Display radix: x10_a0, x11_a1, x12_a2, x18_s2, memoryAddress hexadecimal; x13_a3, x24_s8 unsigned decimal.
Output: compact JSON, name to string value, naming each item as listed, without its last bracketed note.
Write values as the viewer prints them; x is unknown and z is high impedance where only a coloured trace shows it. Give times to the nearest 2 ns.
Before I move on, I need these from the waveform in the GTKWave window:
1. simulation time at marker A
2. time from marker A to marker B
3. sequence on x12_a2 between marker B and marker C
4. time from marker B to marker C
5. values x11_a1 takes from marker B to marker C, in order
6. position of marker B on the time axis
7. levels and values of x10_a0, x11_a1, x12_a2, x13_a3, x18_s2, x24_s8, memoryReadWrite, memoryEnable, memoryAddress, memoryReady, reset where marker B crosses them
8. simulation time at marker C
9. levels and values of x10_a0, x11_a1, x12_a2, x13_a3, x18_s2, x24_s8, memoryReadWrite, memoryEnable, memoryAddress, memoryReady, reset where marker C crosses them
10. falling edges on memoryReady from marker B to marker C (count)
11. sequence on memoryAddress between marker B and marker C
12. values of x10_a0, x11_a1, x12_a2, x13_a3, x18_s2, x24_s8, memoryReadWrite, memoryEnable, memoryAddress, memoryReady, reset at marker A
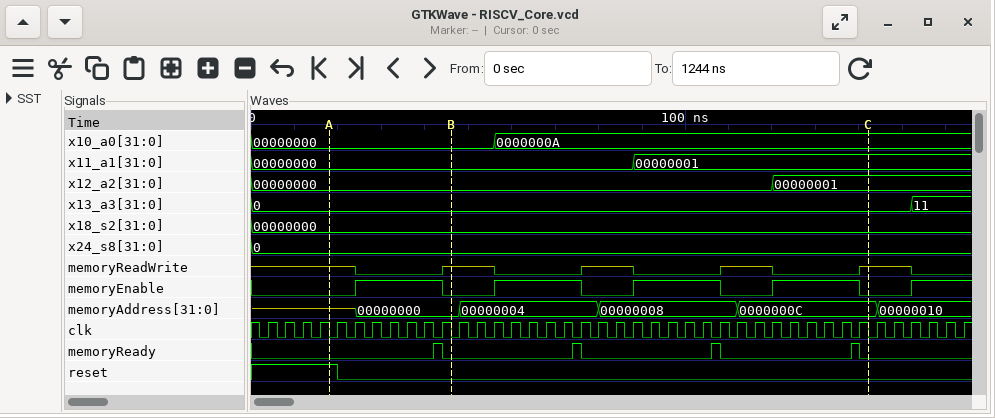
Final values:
{"simulation time at marker A": "18 ns", "time from marker A to marker B": "28 ns", "sequence on x12_a2 between marker B and marker C": "00000000, 00000001", "time from marker B to marker C": "96 ns", "values x11_a1 takes from marker B to marker C, in order": "00000000, 00000001", "position of marker B on the time axis": "46 ns", "levels and values of x10_a0, x11_a1, x12_a2, x13_a3, x18_s2, x24_s8, memoryReadWrite, memoryEnable, memoryAddress, memoryReady, reset where marker B crosses them": "x10_a0=00000000, x11_a1=00000000, x12_a2=00000000, x13_a3=0, x18_s2=00000000, x24_s8=0, memoryReadWrite=z, memoryEnable=0, memoryAddress=00000000, memoryReady=0, reset=0", "simulation time at marker C": "142 ns", "levels and values of x10_a0, x11_a1, x12_a2, x13_a3, x18_s2, x24_s8, memoryReadWrite, memoryEnable, memoryAddress, memoryReady, reset where marker C crosses them": "x10_a0=0000000A, x11_a1=00000001, x12_a2=00000001, x13_a3=0, x18_s2=00000000, x24_s8=0, memoryReadWrite=z, memoryEnable=0, memoryAddress=0000000C, memoryReady=0, reset=0", "falling edges on memoryReady from marker B to marker C": "3", "sequence on memoryAddress between marker B and marker C": "00000000, 00000004, 00000008, 0000000C", "values of x10_a0, x11_a1, x12_a2, x13_a3, x18_s2, x24_s8, memoryReadWrite, memoryEnable, memoryAddress, memoryReady, reset at marker A": "x10_a0=00000000, x11_a1=00000000, x12_a2=00000000, x13_a3=0, x18_s2=00000000, x24_s8=0, memoryReadWrite=z, memoryEnable=0, memoryAddress=z, memoryReady=0, reset=1"}
